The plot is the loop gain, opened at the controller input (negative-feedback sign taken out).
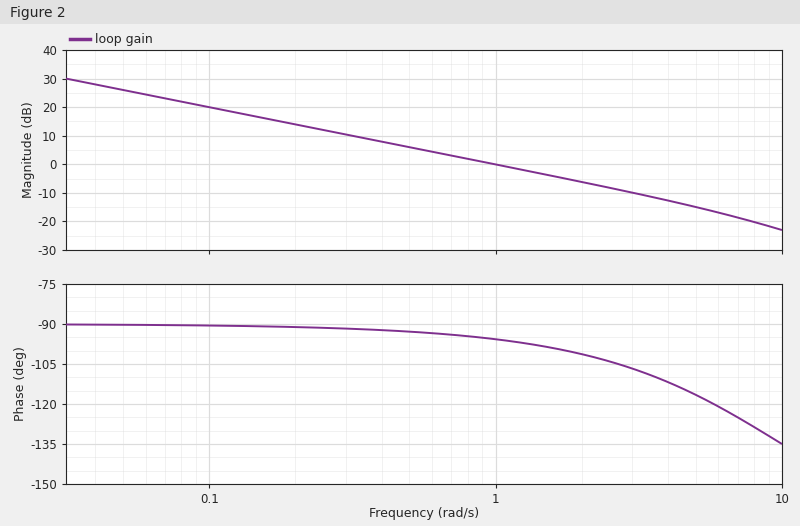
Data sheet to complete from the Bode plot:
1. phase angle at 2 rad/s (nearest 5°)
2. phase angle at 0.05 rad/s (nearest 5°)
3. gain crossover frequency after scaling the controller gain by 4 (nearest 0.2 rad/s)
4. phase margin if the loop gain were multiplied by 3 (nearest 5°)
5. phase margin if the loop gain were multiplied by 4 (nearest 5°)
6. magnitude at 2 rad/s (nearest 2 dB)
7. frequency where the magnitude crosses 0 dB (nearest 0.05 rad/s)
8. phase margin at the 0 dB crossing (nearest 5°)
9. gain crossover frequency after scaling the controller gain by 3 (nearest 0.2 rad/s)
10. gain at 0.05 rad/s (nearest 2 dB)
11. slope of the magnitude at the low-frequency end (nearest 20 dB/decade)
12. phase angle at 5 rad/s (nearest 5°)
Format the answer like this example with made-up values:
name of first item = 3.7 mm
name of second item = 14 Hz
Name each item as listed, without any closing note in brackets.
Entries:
phase angle at 2 rad/s = -100°
phase angle at 0.05 rad/s = -90°
gain crossover frequency after scaling the controller gain by 4 = 3.8 rad/s
phase margin if the loop gain were multiplied by 3 = 75°
phase margin if the loop gain were multiplied by 4 = 70°
magnitude at 2 rad/s = -6 dB
frequency where the magnitude crosses 0 dB = 1.00 rad/s
phase margin at the 0 dB crossing = 85°
gain crossover frequency after scaling the controller gain by 3 = 2.8 rad/s
gain at 0.05 rad/s = 26 dB
slope of the magnitude at the low-frequency end = -20 dB/decade
phase angle at 5 rad/s = -115°
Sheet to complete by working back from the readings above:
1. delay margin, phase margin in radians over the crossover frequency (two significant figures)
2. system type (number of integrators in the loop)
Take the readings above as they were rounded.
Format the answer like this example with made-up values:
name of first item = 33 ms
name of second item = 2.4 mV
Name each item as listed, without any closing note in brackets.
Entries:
delay margin, phase margin in radians over the crossover frequency = 1.5 s
system type = 1
